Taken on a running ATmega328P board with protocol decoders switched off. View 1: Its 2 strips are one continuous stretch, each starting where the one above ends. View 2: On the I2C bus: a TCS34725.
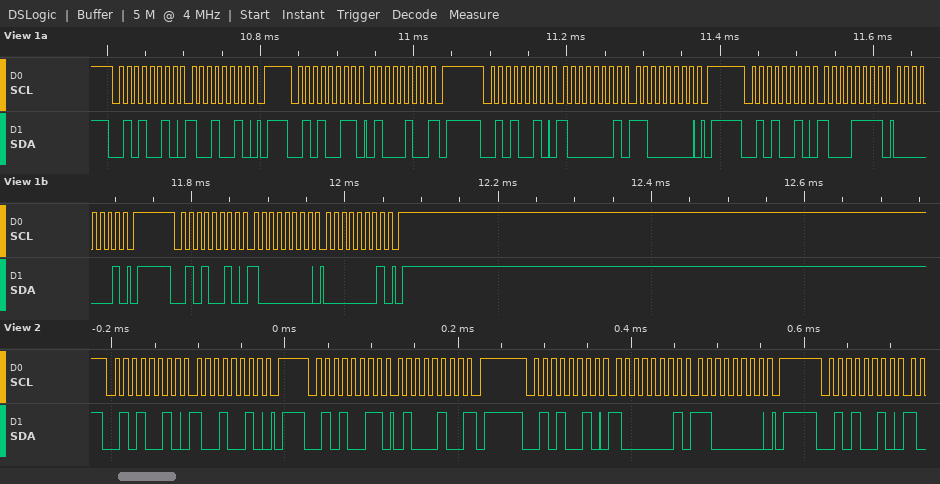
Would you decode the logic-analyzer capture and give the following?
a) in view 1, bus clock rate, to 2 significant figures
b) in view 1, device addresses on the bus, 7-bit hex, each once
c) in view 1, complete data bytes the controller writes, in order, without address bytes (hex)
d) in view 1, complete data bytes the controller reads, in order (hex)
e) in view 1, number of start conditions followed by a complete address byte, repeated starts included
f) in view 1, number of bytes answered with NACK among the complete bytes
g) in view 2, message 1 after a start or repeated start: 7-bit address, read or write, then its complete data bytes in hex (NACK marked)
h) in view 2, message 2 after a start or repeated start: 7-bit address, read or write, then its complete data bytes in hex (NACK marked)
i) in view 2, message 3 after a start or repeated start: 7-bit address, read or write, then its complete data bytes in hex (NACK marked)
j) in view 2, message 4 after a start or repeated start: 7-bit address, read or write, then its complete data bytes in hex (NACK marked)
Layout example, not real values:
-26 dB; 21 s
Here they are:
100 kHz; 0x29; 92 81 C0 8F 01 80 01; 44; 5; 1; 0x29 write: 92; 0x29 read: 44 NACK; 0x29 write: 81 C0; 0x29 write
